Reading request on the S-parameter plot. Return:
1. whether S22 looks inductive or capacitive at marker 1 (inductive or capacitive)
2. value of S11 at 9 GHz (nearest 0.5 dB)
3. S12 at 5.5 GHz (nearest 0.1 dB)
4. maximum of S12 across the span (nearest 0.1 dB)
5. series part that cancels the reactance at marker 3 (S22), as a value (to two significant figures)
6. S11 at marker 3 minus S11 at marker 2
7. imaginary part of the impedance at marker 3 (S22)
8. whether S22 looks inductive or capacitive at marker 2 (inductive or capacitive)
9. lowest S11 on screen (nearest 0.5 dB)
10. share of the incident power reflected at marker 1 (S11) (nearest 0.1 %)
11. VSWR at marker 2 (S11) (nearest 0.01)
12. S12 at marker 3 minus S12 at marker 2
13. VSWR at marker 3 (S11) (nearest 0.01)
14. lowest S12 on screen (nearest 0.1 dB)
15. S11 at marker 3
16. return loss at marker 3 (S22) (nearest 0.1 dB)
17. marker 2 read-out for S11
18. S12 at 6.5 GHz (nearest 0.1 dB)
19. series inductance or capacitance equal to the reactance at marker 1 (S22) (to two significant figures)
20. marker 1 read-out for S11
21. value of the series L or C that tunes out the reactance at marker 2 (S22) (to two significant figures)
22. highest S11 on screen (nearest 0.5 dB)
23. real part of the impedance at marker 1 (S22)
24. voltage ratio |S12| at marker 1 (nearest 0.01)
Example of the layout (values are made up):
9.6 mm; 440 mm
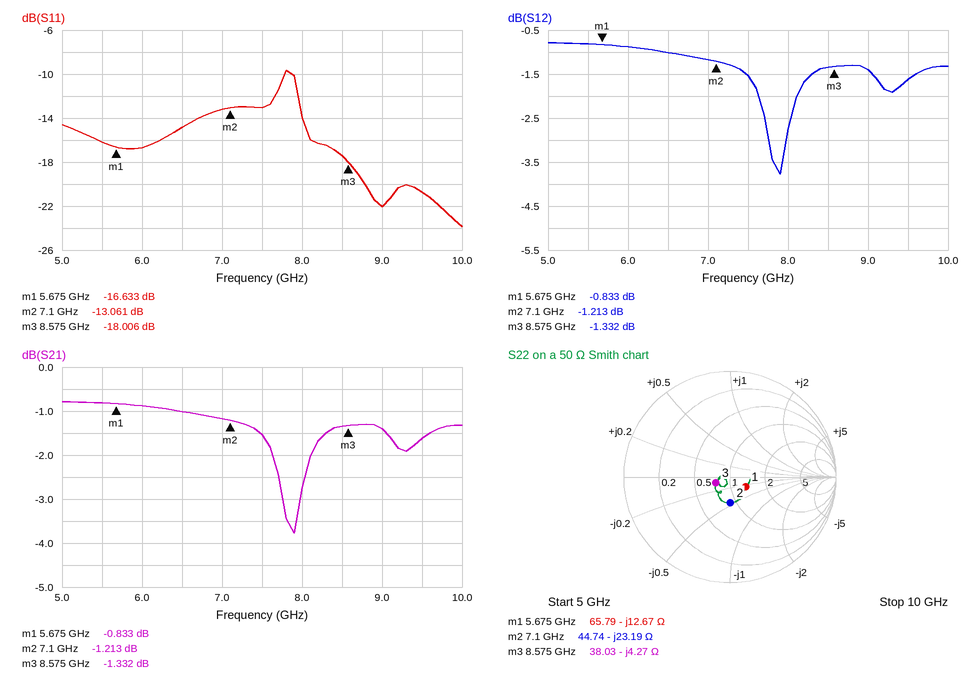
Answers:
capacitive; -22.0 dB; -0.8 dB; -0.8 dB; 79 pH; -4.945 dB; -4.27 Ω; capacitive; -24.0 dB; 2.2 %; 1.57; -0.119 dB; 1.29; -3.8 dB; -18.006 dB; 16.8 dB; -13.061 dB; -1.0 dB; 2.2 pF; -16.633 dB; 520 pH; -9.5 dB; 65.79 Ω; 0.91
